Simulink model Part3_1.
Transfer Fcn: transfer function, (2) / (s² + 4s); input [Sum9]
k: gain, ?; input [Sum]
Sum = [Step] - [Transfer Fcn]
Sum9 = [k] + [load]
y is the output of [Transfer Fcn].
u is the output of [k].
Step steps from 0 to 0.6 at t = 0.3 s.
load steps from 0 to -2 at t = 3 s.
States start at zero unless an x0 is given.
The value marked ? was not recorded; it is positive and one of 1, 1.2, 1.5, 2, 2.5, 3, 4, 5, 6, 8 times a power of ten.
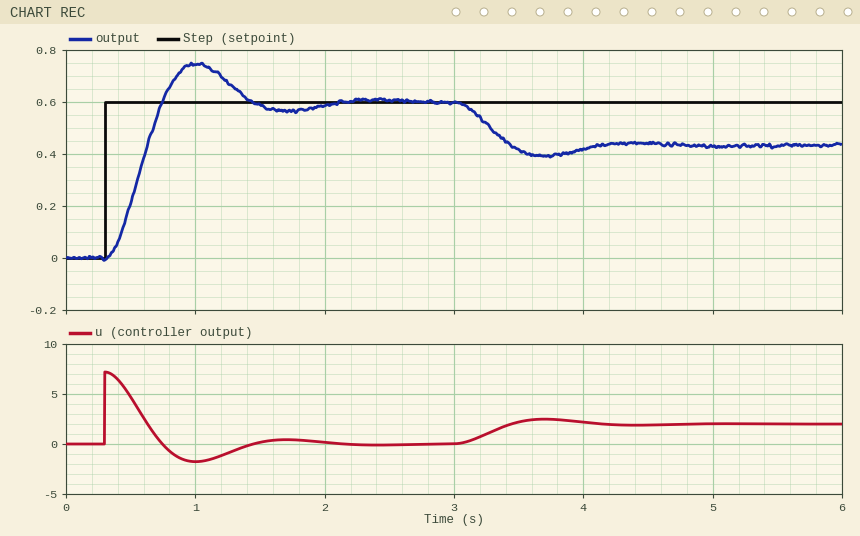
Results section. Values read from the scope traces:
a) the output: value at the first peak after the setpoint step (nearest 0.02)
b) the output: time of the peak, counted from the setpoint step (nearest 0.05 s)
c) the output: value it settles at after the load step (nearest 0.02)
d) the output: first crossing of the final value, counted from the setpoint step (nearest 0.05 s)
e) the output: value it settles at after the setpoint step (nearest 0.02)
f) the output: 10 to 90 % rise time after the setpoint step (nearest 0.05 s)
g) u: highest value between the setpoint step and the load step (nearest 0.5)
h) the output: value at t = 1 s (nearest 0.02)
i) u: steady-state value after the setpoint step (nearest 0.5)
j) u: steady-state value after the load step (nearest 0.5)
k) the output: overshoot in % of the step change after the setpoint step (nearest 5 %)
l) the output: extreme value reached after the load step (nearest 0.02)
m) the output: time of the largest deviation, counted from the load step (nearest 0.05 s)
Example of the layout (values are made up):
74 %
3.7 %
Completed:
0.74
0.70 s
0.44
0.45 s
0.60
0.30 s
7.0
0.74
0.0
2.0
25 %
0.40
0.70 s
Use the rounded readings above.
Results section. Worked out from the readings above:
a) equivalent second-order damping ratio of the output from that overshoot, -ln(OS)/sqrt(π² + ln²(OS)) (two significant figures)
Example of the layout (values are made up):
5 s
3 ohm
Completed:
0.40
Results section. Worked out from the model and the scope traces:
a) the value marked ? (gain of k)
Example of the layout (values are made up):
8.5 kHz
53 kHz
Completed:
12
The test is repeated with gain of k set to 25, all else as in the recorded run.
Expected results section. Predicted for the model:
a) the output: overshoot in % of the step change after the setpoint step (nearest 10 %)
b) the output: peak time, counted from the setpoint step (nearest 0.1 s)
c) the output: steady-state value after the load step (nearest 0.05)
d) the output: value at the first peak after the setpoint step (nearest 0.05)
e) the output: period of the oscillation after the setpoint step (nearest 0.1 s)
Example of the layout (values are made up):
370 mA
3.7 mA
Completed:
40 %
0.5 s
0.50
0.85
0.9 s
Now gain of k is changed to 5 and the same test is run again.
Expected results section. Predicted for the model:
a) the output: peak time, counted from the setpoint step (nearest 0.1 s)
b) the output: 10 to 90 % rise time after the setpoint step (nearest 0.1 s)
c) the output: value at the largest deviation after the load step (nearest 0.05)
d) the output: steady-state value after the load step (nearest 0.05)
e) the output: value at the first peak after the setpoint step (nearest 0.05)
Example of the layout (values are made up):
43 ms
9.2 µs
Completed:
1.3 s
0.6 s
0.15
0.20
0.65
